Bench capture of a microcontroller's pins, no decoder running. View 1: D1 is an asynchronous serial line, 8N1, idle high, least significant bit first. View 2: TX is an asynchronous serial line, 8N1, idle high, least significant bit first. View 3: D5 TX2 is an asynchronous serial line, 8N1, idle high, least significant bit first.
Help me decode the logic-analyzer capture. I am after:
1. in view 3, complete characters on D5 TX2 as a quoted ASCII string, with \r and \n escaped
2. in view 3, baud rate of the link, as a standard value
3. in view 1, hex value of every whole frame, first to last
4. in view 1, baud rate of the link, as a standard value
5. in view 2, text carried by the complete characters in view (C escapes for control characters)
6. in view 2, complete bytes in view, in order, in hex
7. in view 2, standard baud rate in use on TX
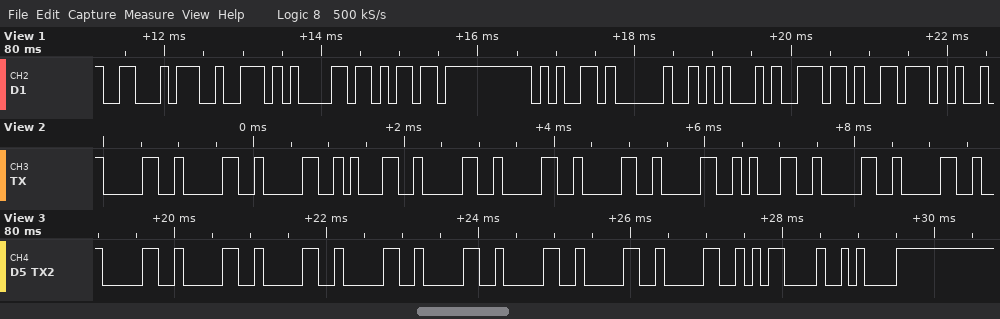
"00000000\r\n"
9600 baud
46 72 61 6D 65 20 45 6E 76
9600 baud
"00010000100"
30 30 30 31 30 30 30 30 31 30 30
9600 baud
